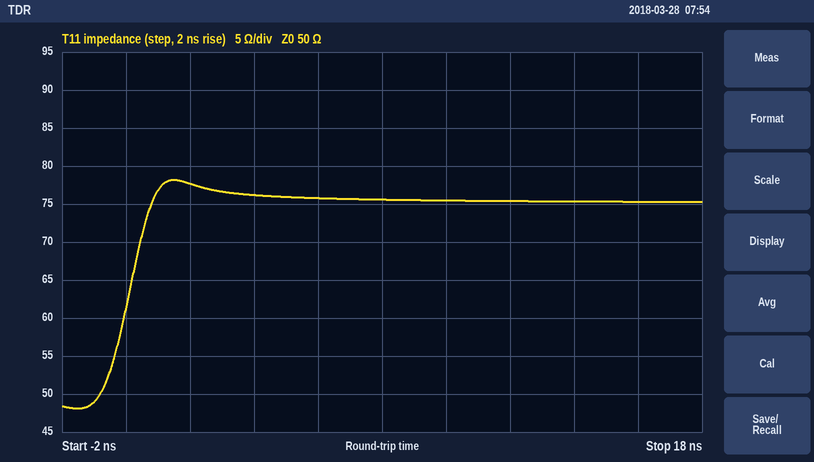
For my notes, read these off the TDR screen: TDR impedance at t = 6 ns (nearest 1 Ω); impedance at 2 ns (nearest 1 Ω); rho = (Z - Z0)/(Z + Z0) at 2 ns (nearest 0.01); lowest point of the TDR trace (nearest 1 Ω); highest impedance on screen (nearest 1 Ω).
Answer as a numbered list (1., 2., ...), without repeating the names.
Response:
1. 76 Ω
2. 78 Ω
3. +0.22
4. 48 Ω
5. 78 Ω
